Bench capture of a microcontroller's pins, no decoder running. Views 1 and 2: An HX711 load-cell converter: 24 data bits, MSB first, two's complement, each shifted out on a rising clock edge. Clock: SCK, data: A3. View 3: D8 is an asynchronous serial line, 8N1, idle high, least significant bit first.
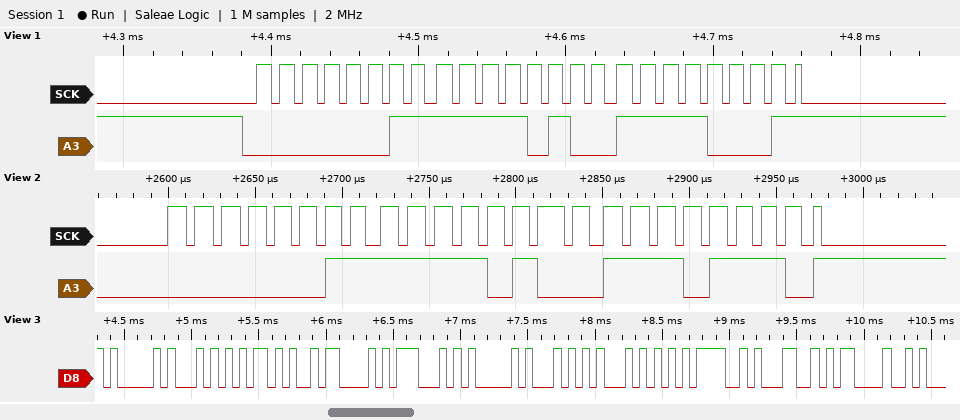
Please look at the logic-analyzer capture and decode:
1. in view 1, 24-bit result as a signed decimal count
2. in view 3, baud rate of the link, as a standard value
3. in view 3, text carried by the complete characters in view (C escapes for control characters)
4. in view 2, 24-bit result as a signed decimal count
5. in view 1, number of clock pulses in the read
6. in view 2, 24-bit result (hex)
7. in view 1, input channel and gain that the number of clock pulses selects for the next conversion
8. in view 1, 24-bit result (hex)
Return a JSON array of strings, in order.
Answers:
["259313", "19200 baud", "\"AT+CGATT=1\\r\"", "259310", "25", "0x03F4EE", "channel A, gain 128", "0x03F4F1"]
